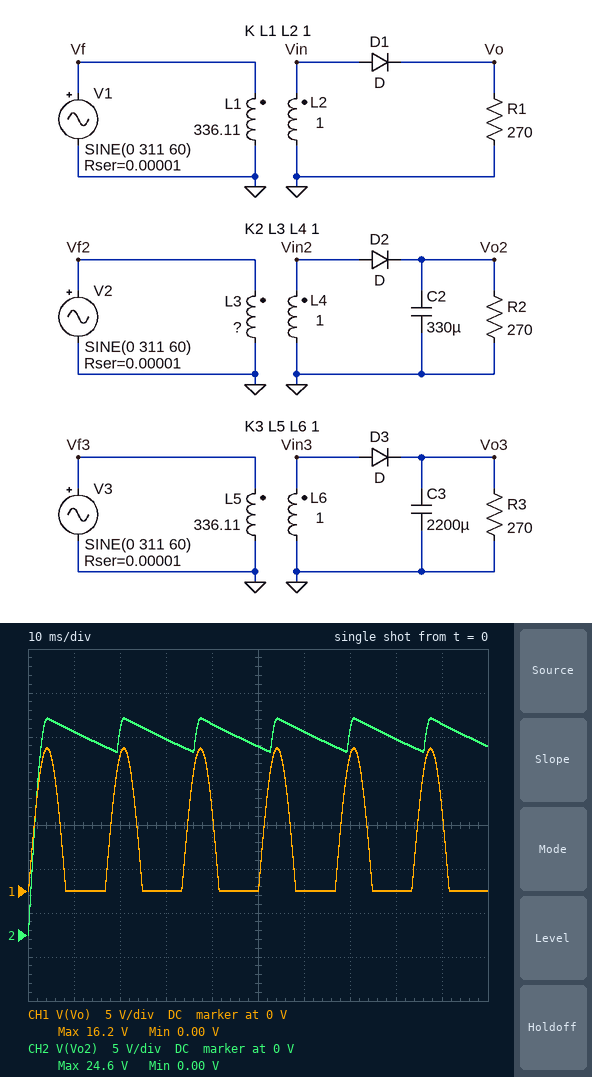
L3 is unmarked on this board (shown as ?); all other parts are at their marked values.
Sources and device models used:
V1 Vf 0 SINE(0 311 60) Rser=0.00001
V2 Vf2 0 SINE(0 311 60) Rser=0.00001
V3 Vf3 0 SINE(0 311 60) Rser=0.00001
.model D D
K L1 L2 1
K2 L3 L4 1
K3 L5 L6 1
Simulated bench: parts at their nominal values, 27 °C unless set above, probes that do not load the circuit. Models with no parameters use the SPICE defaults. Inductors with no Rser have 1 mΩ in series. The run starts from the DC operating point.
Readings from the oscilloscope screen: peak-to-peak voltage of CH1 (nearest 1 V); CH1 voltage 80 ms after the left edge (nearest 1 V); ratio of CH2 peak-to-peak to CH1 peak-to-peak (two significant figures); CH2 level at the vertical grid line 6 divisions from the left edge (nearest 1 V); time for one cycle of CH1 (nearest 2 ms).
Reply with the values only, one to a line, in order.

16 V
0 V
1.5
23 V
16 ms
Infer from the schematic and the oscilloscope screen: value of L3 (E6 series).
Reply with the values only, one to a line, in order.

150 H
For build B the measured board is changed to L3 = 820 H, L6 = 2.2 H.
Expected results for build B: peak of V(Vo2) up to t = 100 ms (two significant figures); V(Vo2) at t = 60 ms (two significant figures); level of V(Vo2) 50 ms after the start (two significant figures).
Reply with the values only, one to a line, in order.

10 V
9.5 V
8.8 V
